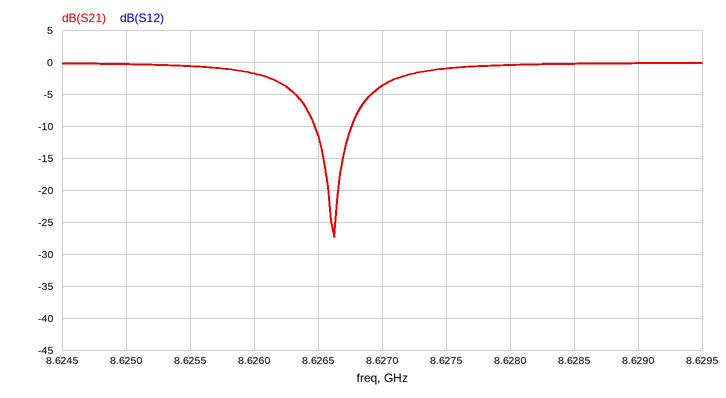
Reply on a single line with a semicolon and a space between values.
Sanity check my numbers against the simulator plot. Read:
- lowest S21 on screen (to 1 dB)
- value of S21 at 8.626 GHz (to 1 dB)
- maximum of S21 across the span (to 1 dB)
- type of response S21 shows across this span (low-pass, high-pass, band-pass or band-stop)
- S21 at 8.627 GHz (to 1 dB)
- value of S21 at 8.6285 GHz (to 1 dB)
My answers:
-27 dB; -2 dB; 0 dB; band-stop; -4 dB; 0 dB
